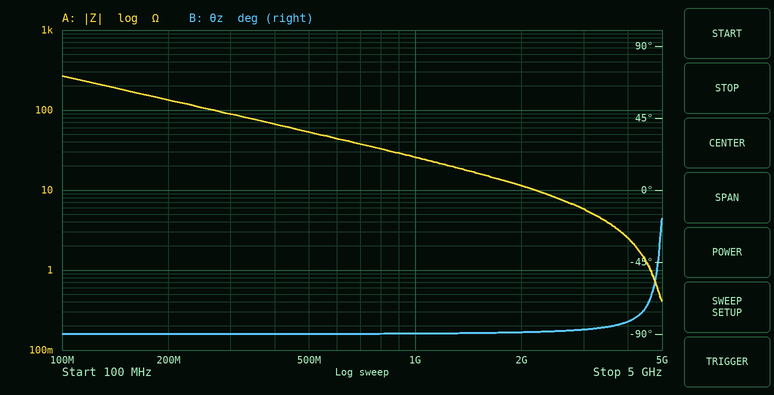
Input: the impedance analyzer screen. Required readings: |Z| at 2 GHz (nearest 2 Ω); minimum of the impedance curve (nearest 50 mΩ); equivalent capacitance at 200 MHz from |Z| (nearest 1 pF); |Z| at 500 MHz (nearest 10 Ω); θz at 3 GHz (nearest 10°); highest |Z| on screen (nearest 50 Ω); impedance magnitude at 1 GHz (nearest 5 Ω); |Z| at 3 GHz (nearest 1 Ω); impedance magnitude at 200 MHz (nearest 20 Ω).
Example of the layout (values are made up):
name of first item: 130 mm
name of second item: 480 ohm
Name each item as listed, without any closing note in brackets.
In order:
|Z| at 2 GHz: 12 Ω
minimum of the impedance curve: 400 mΩ
equivalent capacitance at 200 MHz from |Z|: 6 pF
|Z| at 500 MHz: 50 Ω
θz at 3 GHz: -90°
highest |Z| on screen: 250 Ω
impedance magnitude at 1 GHz: 25 Ω
|Z| at 3 GHz: 6 Ω
impedance magnitude at 200 MHz: 140 Ω
